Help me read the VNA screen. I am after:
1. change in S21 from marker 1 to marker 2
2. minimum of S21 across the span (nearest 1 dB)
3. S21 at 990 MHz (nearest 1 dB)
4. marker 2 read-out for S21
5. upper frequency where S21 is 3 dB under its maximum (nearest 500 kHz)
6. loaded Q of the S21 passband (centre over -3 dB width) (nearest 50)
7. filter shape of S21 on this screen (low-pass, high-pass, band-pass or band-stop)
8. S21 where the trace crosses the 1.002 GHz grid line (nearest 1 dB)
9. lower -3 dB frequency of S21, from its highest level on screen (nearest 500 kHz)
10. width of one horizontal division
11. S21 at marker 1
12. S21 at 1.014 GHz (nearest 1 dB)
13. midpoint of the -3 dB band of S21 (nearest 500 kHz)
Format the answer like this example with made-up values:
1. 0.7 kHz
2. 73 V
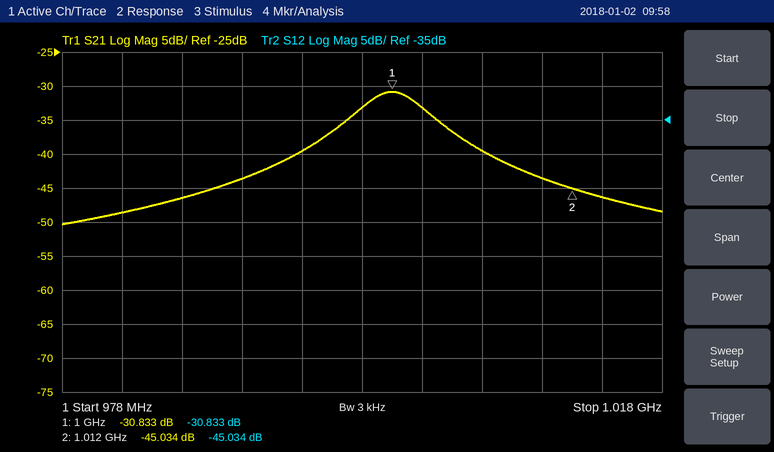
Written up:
1. -14.201 dB
2. -50 dB
3. -44 dB
4. -45.034 dB
5. 1.0025 GHz
6. 200
7. band-pass
8. -33 dB
9. 997.5 MHz
10. 4 MHz
11. -30.833 dB
12. -46 dB
13. 1.0000 GHz
